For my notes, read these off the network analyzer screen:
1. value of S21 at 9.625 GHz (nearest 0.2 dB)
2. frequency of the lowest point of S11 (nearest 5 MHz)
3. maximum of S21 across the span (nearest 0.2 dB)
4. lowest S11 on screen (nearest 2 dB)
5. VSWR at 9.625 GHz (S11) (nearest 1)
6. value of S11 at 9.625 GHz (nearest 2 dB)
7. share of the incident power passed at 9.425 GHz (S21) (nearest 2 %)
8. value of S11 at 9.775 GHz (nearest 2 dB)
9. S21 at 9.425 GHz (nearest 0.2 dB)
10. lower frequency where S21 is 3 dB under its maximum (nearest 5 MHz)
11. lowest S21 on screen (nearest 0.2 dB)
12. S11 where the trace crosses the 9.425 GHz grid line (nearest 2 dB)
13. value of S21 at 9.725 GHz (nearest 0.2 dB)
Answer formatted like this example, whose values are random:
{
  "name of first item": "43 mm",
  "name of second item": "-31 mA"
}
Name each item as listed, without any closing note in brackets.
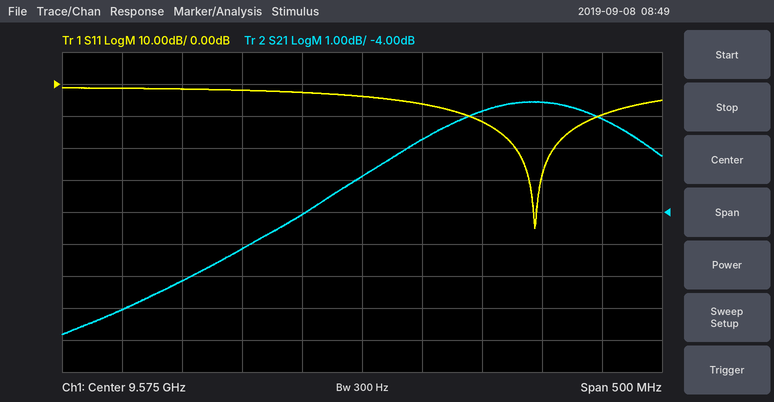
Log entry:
{
  "value of S21 at 9.625 GHz": "-1.8 dB",
  "frequency of the lowest point of S11": "9.720 GHz",
  "maximum of S21 across the span": "-0.6 dB",
  "lowest S11 on screen": "-46 dB",
  "VSWR at 9.625 GHz (S11)": "3",
  "value of S11 at 9.625 GHz": "-6 dB",
  "share of the incident power passed at 9.425 GHz (S21)": "24 %",
  "value of S11 at 9.775 GHz": "-10 dB",
  "S21 at 9.425 GHz": "-6.2 dB",
  "lower frequency where S21 is 3 dB under its maximum": "9.545 GHz",
  "lowest S21 on screen": "-7.8 dB",
  "S11 where the trace crosses the 9.425 GHz grid line": "-2 dB",
  "value of S21 at 9.725 GHz": "-0.6 dB"
}
